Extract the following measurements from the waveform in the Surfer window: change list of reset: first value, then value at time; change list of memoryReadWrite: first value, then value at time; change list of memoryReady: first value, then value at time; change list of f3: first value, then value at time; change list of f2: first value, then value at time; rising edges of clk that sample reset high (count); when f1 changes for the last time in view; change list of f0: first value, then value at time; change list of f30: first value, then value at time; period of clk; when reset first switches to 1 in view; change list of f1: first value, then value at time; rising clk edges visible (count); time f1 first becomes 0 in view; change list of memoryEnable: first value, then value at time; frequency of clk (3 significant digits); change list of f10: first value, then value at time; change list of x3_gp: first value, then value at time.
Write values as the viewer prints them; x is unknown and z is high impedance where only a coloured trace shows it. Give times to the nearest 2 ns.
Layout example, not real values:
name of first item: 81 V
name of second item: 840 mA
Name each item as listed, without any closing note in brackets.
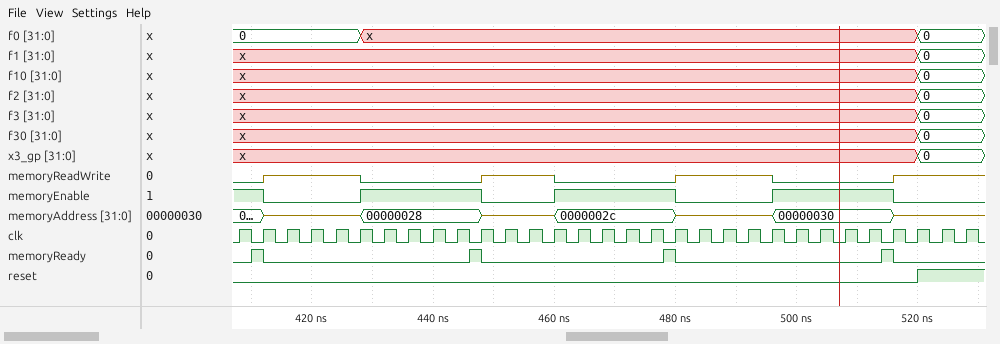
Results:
change list of reset: first value, then value at time: 0, 1 at 520 ns
change list of memoryReadWrite: first value, then value at time: 0, z at 412 ns, 0 at 428 ns, z at 448 ns, 0 at 460 ns, z at 480 ns, 0 at 496 ns, z at 516 ns
change list of memoryReady: first value, then value at time: 0, 1 at 410 ns, 0 at 412 ns, 1 at 446 ns, 0 at 448 ns, 1 at 478 ns, 0 at 480 ns, 1 at 514 ns, 0 at 516 ns
change list of f3: first value, then value at time: x, 0 at 520 ns
change list of f2: first value, then value at time: x, 0 at 520 ns
rising edges of clk that sample reset high: 2
when f1 changes for the last time in view: 520 ns
change list of f0: first value, then value at time: 0, x at 428 ns, 0 at 520 ns
change list of f30: first value, then value at time: x, 0 at 520 ns
period of clk: 4 ns
when reset first switches to 1 in view: 520 ns
change list of f1: first value, then value at time: x, 0 at 520 ns
rising clk edges visible: 31
time f1 first becomes 0 in view: 520 ns
change list of memoryEnable: first value, then value at time: 1, 0 at 412 ns, 1 at 428 ns, 0 at 448 ns, 1 at 460 ns, 0 at 480 ns, 1 at 496 ns, 0 at 516 ns
frequency of clk: 250 MHz
change list of f10: first value, then value at time: x, 0 at 520 ns
change list of x3_gp: first value, then value at time: x, 0 at 520 ns
